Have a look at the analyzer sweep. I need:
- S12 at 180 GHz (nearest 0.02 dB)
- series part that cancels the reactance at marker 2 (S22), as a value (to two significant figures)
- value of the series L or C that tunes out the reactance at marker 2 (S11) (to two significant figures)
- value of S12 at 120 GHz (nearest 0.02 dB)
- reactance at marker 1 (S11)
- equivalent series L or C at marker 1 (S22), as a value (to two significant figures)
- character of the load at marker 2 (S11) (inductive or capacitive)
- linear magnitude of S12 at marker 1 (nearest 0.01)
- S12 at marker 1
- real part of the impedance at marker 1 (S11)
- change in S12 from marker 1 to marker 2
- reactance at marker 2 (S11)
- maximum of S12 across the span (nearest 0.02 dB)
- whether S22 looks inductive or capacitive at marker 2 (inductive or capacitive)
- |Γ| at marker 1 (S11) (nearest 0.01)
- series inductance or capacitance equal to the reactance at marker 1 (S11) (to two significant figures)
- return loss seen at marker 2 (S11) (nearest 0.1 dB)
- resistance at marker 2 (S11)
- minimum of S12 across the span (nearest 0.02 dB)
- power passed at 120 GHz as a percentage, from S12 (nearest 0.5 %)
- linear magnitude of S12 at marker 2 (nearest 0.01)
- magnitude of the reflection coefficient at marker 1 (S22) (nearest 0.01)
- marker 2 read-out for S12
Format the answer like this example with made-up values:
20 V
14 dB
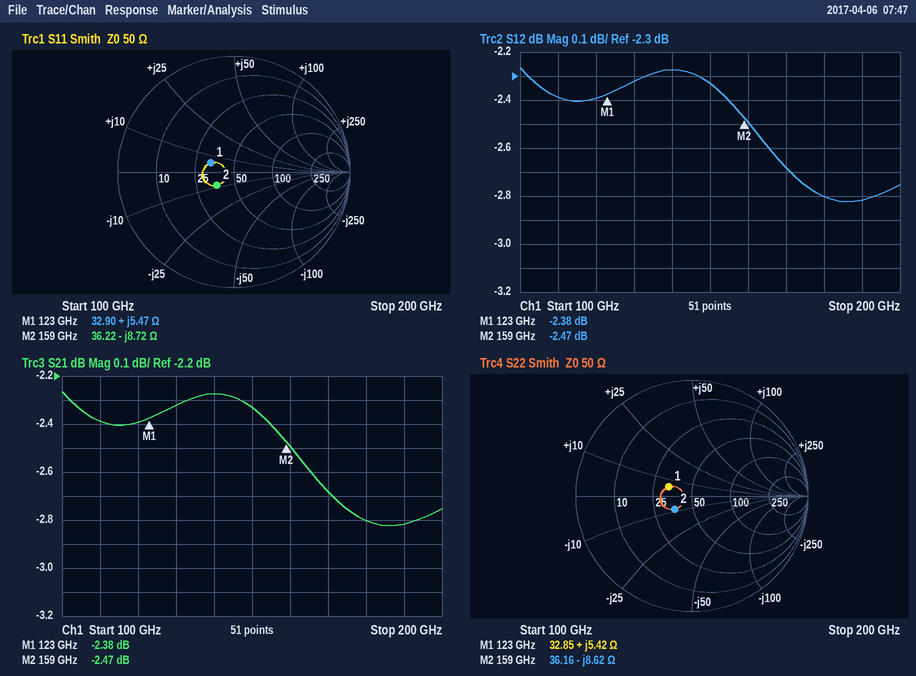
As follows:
-2.80 dB
8.6 pH
8.7 pH
-2.40 dB
+5.47 Ω
7.0 pH
capacitive
0.76
-2.38 dB
32.90 Ω
-0.09 dB
-8.72 Ω
-2.26 dB
capacitive
0.22
7.1 pH
14.5 dB
36.22 Ω
-2.82 dB
57.5 %
0.75
0.22
-2.47 dB
